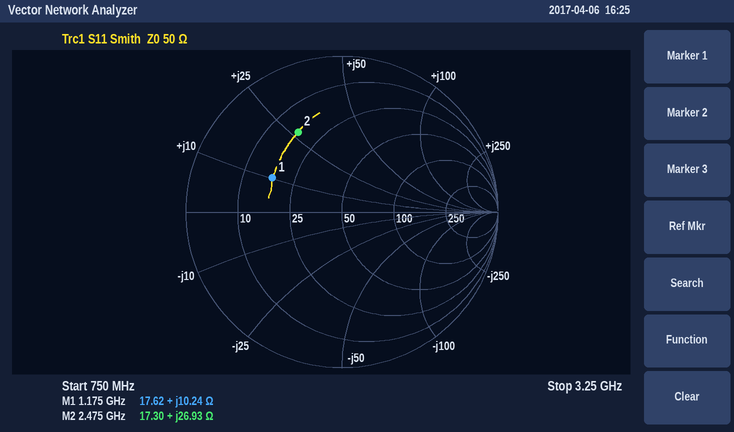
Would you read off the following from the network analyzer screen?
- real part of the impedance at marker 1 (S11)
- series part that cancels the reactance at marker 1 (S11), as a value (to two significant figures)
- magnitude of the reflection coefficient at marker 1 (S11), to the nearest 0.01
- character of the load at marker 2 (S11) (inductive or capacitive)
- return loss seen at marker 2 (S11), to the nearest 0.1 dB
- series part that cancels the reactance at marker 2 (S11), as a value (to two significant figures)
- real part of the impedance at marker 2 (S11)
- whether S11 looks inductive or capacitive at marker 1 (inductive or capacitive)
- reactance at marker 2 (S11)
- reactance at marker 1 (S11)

17.62 Ω
13 pF
0.50
inductive
4.7 dB
2.4 pF
17.30 Ω
inductive
+26.93 Ω
+10.24 Ω
